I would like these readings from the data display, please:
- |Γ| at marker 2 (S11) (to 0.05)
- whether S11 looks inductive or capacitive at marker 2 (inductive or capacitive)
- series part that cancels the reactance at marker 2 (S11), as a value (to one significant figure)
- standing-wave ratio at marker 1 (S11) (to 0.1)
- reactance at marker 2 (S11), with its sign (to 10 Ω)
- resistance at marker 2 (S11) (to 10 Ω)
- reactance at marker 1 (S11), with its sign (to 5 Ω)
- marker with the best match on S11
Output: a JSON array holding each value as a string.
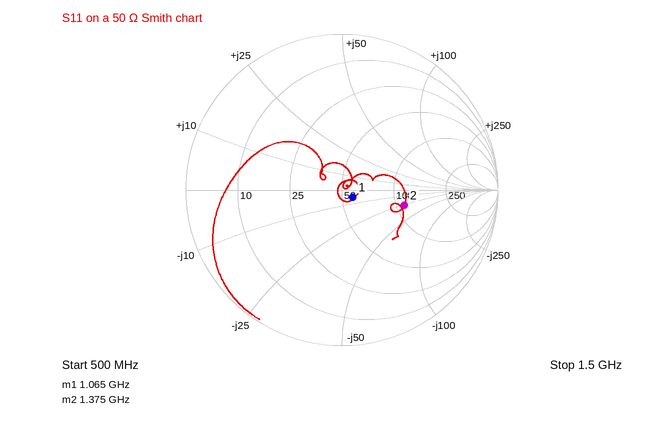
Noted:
["0.40", "capacitive", "3 nH", "1.2", "-30 Ω", "110 Ω", "-5 Ω", "marker 1"]
